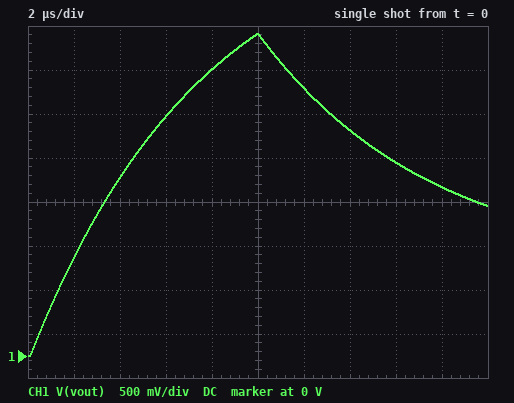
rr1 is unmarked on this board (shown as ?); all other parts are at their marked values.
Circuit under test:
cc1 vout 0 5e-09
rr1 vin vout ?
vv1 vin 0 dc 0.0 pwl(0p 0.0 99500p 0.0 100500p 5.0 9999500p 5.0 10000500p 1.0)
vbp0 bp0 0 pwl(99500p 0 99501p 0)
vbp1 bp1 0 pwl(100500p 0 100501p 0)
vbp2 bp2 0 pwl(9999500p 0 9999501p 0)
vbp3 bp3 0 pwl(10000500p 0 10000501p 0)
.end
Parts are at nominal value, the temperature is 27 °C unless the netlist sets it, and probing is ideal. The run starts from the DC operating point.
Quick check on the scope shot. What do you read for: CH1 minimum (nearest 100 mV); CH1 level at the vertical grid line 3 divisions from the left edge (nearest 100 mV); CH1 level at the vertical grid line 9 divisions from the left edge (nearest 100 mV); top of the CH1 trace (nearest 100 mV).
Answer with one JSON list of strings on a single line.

["0 V", "2.7 V", "1.9 V", "3.7 V"]
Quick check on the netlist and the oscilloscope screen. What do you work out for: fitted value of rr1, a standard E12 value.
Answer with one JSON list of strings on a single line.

["1.5 kΩ"]
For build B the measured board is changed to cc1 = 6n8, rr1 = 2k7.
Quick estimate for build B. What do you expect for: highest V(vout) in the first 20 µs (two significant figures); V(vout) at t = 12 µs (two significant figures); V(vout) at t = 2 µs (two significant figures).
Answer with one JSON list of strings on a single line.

["2.1 V", "2.0 V", "490 mV"]
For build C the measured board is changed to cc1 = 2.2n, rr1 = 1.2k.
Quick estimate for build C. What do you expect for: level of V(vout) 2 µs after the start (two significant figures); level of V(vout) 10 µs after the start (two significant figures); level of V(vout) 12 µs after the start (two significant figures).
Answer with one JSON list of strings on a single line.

["2.6 V", "4.9 V", "2.8 V"]
